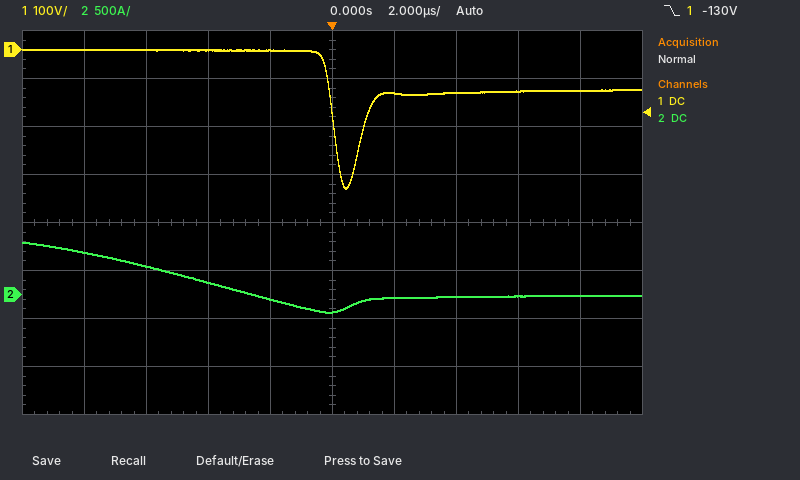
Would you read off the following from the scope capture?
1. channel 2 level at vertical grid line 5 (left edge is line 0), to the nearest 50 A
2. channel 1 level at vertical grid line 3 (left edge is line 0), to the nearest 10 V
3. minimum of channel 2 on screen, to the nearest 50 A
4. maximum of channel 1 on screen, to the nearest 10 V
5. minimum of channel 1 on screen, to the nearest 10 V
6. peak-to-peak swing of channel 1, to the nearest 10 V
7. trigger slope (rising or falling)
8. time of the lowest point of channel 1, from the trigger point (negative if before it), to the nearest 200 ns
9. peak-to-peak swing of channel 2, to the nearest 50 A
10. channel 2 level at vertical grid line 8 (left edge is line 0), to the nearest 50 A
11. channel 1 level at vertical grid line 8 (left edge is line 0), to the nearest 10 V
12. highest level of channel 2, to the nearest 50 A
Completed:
-200 A
0 V
-200 A
0 V
-290 V
290 V
falling
+400 ns
750 A
0 A
-90 V
550 A
